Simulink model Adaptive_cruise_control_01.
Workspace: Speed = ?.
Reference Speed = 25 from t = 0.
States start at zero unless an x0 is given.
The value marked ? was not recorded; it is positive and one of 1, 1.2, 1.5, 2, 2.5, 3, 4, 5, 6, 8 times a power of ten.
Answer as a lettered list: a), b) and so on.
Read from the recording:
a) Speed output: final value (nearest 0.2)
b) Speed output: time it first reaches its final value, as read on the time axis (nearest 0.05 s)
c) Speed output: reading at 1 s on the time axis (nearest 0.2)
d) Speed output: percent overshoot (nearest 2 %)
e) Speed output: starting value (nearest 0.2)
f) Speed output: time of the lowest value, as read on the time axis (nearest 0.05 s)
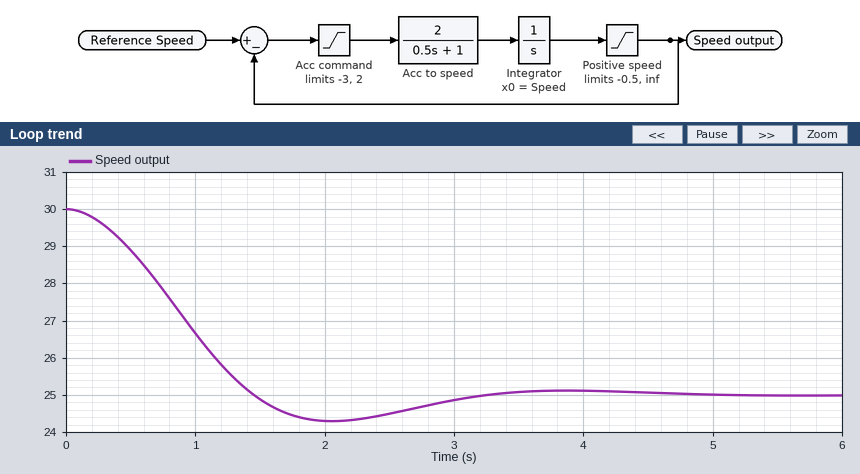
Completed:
a) 25.0
b) 1.45 s
c) 26.6
d) 14 %
e) 30.0
f) 2.05 s
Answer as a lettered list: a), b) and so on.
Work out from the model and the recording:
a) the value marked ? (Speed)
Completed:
a) 30
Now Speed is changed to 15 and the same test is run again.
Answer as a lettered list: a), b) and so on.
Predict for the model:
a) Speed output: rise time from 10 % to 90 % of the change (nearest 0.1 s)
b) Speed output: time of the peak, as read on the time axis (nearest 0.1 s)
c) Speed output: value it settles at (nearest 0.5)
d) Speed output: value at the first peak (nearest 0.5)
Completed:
a) 2.2 s
b) 3.7 s
c) 25.0
d) 25.5
